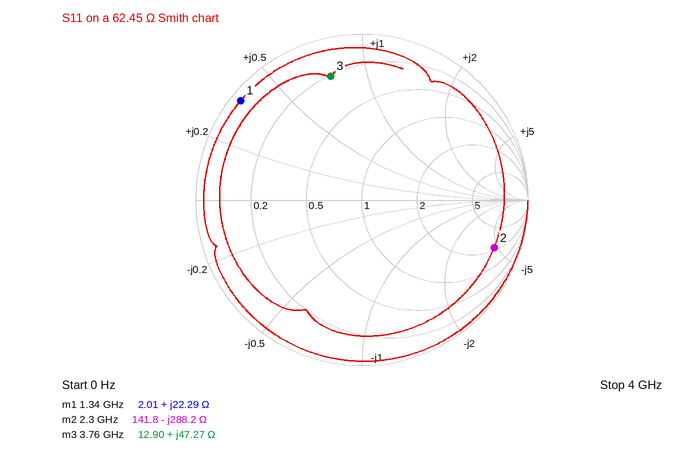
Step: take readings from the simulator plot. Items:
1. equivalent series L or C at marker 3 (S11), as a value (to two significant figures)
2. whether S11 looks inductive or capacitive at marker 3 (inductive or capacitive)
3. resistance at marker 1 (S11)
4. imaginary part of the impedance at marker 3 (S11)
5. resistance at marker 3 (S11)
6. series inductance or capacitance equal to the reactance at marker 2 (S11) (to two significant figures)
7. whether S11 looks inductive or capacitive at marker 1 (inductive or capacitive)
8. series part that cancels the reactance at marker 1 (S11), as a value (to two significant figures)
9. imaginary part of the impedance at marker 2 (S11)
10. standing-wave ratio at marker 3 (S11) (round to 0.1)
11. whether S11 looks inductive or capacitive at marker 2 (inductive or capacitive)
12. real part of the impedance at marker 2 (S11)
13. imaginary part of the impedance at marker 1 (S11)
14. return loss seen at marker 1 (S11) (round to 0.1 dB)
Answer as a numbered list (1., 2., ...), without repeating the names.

1. 2.0 nH
2. inductive
3. 2.01 Ω
4. +47.27 Ω
5. 12.90 Ω
6. 240 fF
7. inductive
8. 5.3 pF
9. -288.2 Ω
10. 7.7
11. capacitive
12. 141.8 Ω
13. +22.29 Ω
14. 0.5 dB
